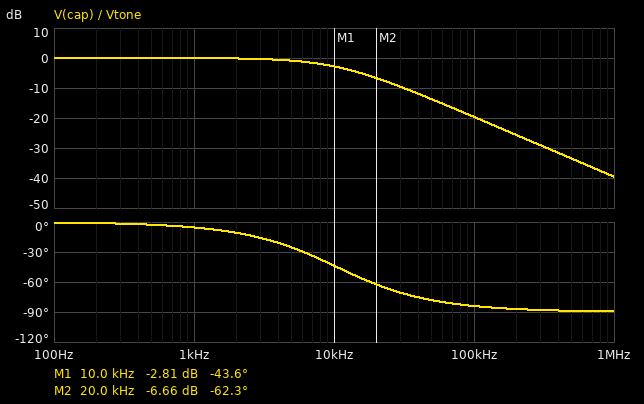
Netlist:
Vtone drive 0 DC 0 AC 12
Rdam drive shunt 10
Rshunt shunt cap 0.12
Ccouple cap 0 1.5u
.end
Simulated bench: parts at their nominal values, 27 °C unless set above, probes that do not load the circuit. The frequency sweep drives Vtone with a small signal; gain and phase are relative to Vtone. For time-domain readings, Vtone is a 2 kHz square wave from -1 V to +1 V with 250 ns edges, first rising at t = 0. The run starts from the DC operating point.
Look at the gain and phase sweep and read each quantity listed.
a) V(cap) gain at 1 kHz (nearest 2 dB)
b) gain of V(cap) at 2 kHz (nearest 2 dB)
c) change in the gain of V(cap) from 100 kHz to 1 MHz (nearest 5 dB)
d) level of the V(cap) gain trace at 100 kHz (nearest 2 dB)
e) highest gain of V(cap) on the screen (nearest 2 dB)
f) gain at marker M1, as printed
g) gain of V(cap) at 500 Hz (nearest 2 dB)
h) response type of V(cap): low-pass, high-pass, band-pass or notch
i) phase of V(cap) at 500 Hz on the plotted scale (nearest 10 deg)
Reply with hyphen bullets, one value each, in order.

- 0 dB
- 0 dB
- -20 dB
- -20 dB
- 0 dB
- -2.81 dB
- 0 dB
- low-pass
- 0 deg
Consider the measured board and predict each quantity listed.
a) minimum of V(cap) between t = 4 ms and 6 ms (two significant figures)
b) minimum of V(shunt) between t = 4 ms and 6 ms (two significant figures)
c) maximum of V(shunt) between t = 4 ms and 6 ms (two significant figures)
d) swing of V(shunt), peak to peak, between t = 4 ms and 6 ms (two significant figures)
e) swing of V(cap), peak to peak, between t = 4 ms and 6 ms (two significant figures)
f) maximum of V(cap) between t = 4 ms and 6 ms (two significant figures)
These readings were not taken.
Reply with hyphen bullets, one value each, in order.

- -1.0 V
- -1.0 V
- 1.0 V
- 2.0 V
- 2.0 V
- 1.0 V
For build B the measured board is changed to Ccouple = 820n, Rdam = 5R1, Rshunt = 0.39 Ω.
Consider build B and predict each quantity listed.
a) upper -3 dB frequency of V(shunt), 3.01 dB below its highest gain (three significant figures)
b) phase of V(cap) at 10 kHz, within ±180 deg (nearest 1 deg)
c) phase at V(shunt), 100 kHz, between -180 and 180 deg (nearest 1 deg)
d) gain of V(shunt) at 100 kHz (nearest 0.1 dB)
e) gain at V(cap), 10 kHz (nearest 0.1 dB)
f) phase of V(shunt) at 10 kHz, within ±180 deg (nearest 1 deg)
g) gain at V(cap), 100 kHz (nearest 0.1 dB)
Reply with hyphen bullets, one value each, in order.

- 35.5 kHz
- -16 deg
- -59 deg
- -9.4 dB
- -0.3 dB
- -15 deg
- -9.5 dB
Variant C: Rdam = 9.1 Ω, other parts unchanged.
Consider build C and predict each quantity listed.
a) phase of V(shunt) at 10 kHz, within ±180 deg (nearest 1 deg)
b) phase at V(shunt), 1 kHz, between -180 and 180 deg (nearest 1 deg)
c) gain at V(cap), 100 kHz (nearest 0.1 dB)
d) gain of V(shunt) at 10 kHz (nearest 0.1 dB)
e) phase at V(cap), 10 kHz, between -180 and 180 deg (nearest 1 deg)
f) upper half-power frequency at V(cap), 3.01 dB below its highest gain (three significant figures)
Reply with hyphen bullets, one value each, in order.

- -40 deg
- -5 deg
- -18.8 dB
- -2.4 dB
- -41 deg
- 11.5 kHz
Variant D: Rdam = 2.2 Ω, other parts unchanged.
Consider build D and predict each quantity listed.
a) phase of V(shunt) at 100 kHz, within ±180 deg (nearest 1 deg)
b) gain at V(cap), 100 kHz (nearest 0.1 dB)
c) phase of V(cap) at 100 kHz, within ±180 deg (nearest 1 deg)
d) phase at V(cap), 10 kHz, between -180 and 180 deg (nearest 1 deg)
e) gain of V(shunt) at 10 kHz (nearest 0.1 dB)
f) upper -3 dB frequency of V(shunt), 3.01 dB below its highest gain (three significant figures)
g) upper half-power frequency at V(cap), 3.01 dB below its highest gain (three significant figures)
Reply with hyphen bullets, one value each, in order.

- -59 deg
- -7.6 dB
- -65 deg
- -12 deg
- -0.2 dB
- 45.9 kHz
- 45.7 kHz
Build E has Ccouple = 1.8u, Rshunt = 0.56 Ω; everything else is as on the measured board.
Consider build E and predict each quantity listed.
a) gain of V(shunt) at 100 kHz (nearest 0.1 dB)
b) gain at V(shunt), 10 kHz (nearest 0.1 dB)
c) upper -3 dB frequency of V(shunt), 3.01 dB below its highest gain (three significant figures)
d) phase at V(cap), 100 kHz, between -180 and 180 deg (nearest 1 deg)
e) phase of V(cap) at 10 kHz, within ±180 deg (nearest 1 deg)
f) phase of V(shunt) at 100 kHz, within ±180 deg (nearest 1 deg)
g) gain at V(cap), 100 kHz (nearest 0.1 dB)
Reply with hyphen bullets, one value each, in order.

- -20.1 dB
- -3.8 dB
- 8.40 kHz
- -85 deg
- -50 deg
- -53 deg
- -21.6 dB
